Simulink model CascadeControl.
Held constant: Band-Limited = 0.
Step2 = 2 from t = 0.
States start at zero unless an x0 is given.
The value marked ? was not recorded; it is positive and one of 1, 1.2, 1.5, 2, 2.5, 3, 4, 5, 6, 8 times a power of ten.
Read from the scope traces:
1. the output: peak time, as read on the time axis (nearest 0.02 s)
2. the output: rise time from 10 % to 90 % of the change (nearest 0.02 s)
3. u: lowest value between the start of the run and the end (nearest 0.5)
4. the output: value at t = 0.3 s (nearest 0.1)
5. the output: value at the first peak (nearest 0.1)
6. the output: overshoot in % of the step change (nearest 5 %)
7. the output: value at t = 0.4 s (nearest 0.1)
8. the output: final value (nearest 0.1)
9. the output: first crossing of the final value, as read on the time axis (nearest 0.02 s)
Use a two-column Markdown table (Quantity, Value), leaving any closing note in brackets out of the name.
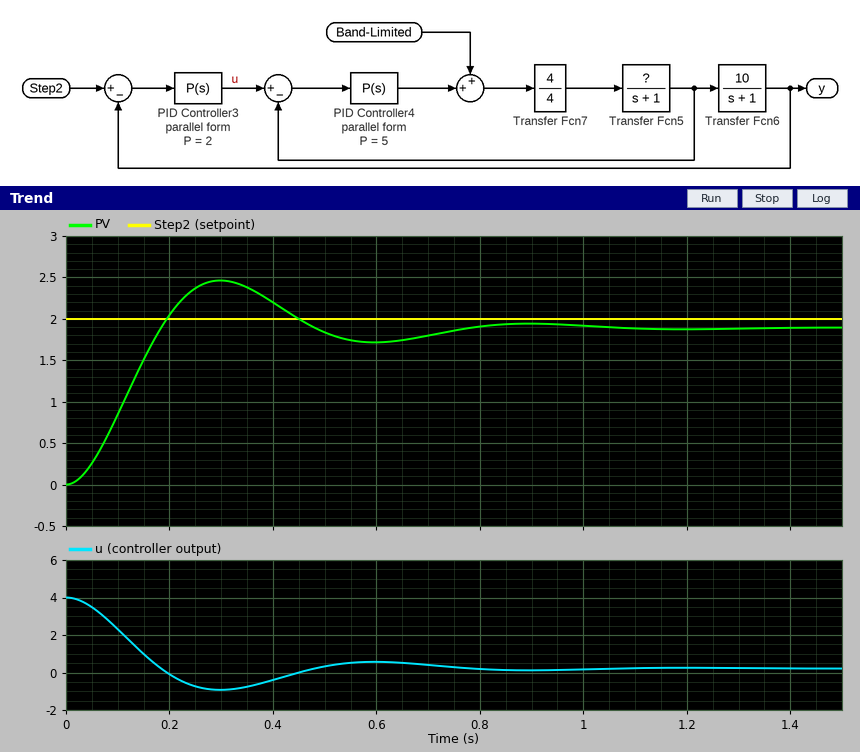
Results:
| Quantity | Value |
|---|---|
| the output: peak time, as read on the time axis | 0.30 s |
| the output: rise time from 10 % to 90 % of the change | 0.12 s |
| u: lowest value between the start of the run and the end | -1.0 |
| the output: value at t = 0.3 s | 2.5 |
| the output: value at the first peak | 2.5 |
| the output: overshoot in % of the step change | 30 % |
| the output: value at t = 0.4 s | 2.2 |
| the output: final value | 1.9 |
| the output: first crossing of the final value, as read on the time axis | 0.18 s |
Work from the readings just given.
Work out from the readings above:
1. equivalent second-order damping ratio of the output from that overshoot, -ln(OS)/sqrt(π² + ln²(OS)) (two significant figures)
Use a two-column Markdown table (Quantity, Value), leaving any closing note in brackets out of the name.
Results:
| Quantity | Value |
|---|---|
| equivalent second-order damping ratio of the output from that overshoot, -ln(OS)/sqrt(π² + ln²(OS)) | 0.36 |
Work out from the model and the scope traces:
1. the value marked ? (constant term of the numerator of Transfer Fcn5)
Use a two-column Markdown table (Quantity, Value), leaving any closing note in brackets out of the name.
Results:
| Quantity | Value |
|---|---|
| the value marked ? | 1.2 |
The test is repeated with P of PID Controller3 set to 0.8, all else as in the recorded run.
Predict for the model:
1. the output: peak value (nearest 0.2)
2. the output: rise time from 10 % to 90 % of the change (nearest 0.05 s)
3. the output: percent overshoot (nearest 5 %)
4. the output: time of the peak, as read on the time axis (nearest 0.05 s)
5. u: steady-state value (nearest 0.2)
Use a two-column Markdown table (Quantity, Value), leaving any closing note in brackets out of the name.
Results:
| Quantity | Value |
|---|---|
| the output: peak value | 2.0 |
| the output: rise time from 10 % to 90 % of the change | 0.25 s |
| the output: percent overshoot | 15 % |
| the output: time of the peak, as read on the time axis | 0.50 s |
| u: steady-state value | 0.2 |
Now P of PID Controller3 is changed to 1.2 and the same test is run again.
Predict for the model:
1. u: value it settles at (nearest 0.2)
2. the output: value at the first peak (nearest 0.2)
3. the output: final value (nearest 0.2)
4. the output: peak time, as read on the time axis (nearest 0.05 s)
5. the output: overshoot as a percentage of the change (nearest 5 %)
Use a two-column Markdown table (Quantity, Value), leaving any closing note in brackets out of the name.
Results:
| Quantity | Value |
|---|---|
| u: value it settles at | 0.2 |
| the output: value at the first peak | 2.2 |
| the output: final value | 1.8 |
| the output: peak time, as read on the time axis | 0.40 s |
| the output: overshoot as a percentage of the change | 20 % |
